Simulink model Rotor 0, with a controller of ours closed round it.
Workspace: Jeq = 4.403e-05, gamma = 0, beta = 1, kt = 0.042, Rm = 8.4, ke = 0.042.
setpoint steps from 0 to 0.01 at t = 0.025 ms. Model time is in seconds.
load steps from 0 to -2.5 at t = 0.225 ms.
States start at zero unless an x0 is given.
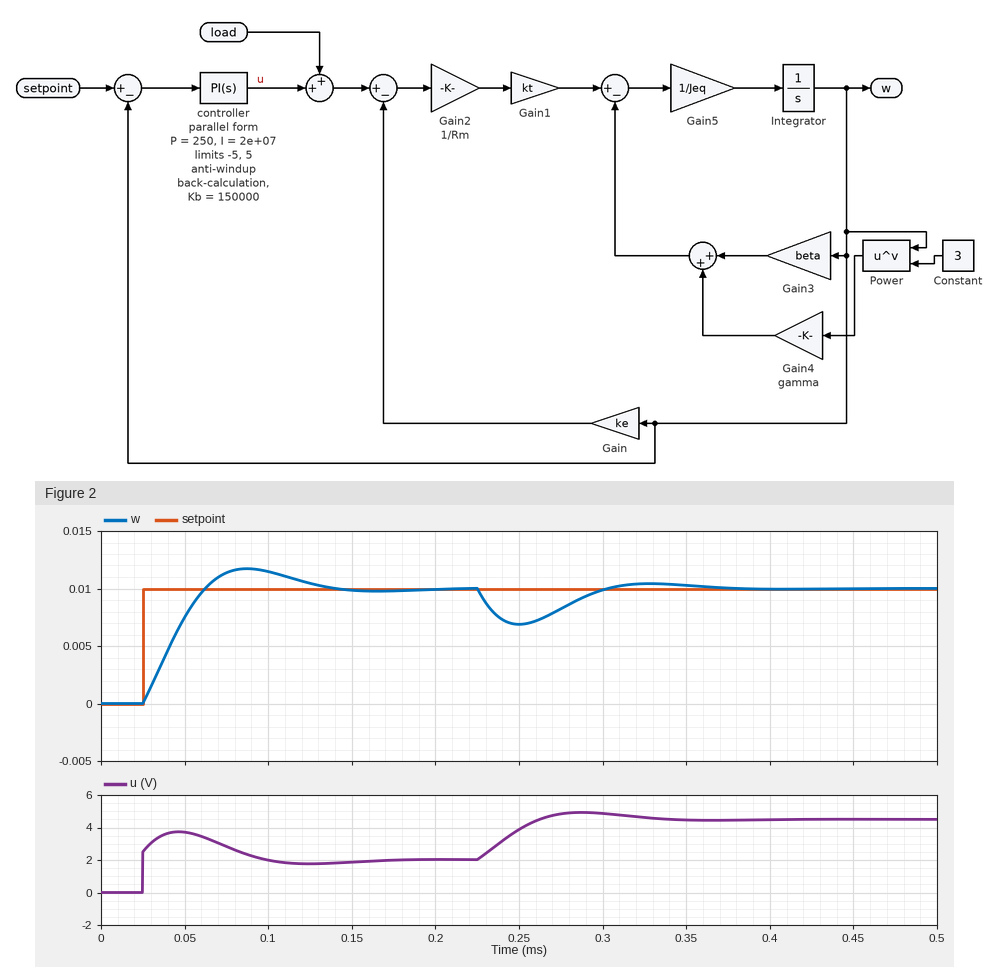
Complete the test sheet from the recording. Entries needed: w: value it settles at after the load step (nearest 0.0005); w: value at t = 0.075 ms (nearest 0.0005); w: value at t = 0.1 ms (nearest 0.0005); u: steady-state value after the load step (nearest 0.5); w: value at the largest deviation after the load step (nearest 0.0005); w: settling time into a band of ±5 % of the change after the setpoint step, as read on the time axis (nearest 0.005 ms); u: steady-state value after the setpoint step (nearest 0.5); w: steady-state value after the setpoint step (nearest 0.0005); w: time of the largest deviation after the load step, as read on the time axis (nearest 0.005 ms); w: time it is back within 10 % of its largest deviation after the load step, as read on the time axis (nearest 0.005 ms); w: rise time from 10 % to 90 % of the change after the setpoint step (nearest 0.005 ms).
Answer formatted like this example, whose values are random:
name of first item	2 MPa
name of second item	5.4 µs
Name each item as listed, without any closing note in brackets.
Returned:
w: value it settles at after the load step	0.0100
w: value at t = 0.075 ms	0.0115
w: value at t = 0.1 ms	0.0115
u: steady-state value after the load step	4.5
w: value at the largest deviation after the load step	0.0070
w: settling time into a band of ±5 % of the change after the setpoint step, as read on the time axis	0.125 ms
u: steady-state value after the setpoint step	2.0
w: steady-state value after the setpoint step	0.0100
w: time of the largest deviation after the load step, as read on the time axis	0.250 ms
w: time it is back within 10 % of its largest deviation after the load step, as read on the time axis	0.345 ms
w: rise time from 10 % to 90 % of the change after the setpoint step	0.030 ms
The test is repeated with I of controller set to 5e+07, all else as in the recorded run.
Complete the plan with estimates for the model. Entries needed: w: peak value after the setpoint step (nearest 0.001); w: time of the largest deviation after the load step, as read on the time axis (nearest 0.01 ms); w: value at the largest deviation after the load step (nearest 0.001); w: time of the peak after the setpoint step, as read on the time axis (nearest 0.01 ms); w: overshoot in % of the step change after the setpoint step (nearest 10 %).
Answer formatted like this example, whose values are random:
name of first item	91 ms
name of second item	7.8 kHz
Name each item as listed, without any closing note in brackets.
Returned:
w: peak value after the setpoint step	0.013
w: time of the largest deviation after the load step, as read on the time axis	0.24 ms
w: value at the largest deviation after the load step	0.008
w: time of the peak after the setpoint step, as read on the time axis	0.07 ms
w: overshoot in % of the step change after the setpoint step	30 %
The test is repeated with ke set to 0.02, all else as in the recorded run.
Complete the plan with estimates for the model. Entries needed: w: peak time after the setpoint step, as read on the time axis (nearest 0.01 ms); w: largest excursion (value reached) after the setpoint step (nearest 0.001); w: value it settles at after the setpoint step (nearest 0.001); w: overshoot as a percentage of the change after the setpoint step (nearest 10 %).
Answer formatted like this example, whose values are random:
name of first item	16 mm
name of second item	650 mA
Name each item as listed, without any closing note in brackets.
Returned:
w: peak time after the setpoint step, as read on the time axis	0.09 ms
w: largest excursion (value reached) after the setpoint step	0.012
w: value it settles at after the setpoint step	0.010
w: overshoot as a percentage of the change after the setpoint step	20 %
